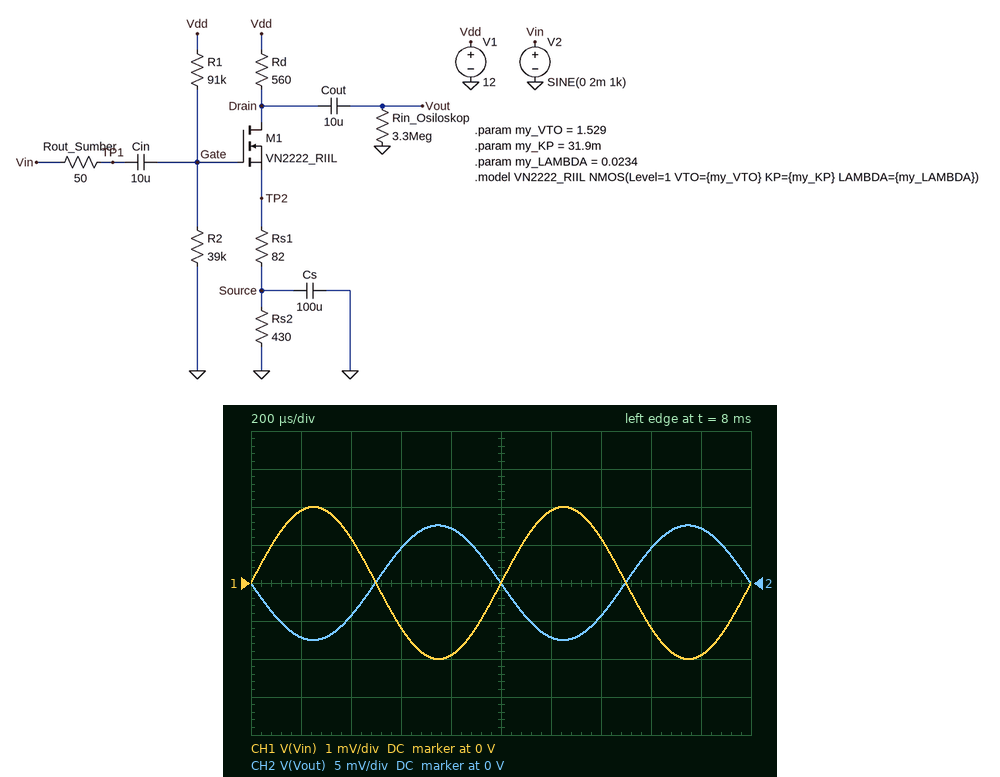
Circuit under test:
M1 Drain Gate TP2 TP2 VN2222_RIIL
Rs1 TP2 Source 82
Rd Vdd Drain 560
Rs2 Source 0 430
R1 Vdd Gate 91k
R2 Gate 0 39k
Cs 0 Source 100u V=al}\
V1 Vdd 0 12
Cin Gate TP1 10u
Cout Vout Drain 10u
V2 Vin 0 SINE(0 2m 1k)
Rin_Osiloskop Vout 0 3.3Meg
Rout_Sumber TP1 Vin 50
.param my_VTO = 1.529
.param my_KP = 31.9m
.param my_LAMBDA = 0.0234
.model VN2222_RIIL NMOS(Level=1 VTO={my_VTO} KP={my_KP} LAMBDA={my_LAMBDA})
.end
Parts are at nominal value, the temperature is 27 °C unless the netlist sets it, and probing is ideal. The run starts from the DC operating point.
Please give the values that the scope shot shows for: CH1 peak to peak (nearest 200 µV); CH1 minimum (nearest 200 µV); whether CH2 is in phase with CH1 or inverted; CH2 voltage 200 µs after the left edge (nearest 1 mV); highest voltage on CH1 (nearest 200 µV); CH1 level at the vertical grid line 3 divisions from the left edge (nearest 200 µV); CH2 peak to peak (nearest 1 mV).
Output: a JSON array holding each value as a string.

["4.0 mV", "-2.0 mV", "inverted", "-7 mV", "2.0 mV", "-1.2 mV", "15 mV"]
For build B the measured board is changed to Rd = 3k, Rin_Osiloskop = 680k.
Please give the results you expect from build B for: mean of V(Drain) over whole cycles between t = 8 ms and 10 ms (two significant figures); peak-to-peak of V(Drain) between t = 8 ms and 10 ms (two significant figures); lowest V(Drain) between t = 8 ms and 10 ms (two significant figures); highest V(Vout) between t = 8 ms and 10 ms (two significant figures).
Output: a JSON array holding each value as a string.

["2.5 V", "71 mV", "2.4 V", "36 mV"]
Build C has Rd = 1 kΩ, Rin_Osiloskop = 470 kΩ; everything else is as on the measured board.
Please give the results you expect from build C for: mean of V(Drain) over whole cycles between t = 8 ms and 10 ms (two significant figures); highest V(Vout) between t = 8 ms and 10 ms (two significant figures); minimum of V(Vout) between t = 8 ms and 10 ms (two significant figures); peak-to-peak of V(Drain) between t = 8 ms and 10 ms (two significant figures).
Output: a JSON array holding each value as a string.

["8.8 V", "13 mV", "-13 mV", "26 mV"]
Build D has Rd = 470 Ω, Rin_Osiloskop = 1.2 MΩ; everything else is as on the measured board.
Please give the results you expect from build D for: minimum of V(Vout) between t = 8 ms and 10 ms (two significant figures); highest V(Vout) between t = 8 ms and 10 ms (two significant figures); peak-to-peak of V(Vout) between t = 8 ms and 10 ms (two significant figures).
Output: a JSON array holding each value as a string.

["-6.3 mV", "6.4 mV", "13 mV"]
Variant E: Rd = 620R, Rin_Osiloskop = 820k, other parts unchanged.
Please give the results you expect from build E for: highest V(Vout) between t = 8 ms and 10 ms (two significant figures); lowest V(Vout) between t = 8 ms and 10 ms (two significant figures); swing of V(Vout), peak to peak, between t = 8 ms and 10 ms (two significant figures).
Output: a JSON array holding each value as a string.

["8.4 mV", "-8.3 mV", "17 mV"]
